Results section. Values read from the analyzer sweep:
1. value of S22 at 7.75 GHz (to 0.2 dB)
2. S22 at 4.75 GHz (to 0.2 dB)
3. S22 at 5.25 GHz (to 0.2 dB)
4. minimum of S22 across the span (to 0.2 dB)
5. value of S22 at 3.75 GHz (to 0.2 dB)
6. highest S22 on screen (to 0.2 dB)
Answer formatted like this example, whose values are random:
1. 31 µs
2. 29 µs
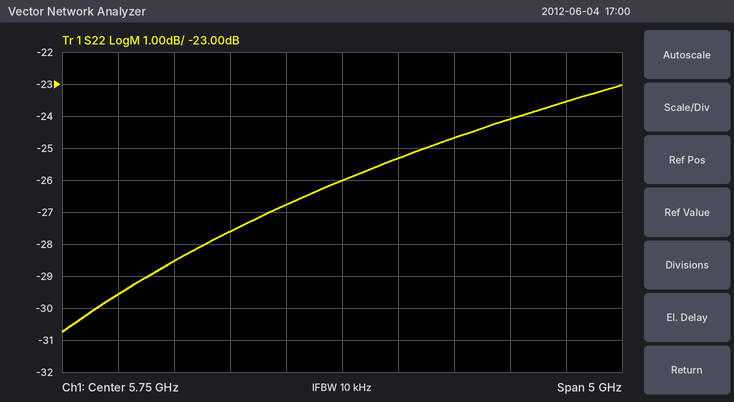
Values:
1. -23.6 dB
2. -27.6 dB
3. -26.8 dB
4. -30.8 dB
5. -29.6 dB
6. -23.0 dB
